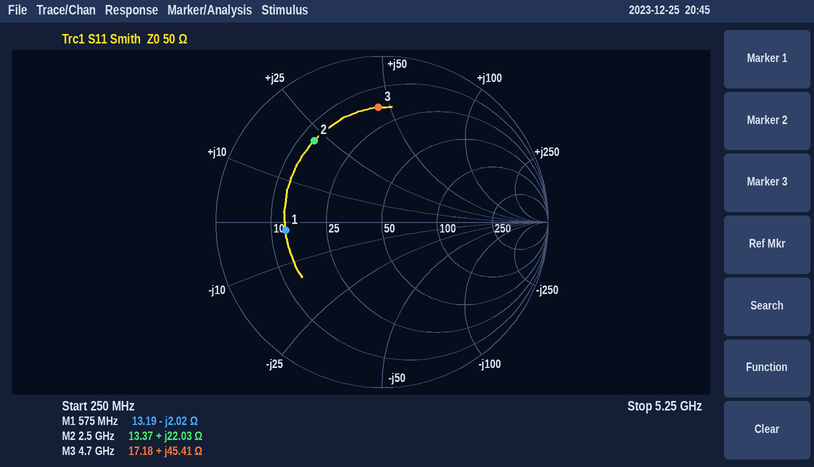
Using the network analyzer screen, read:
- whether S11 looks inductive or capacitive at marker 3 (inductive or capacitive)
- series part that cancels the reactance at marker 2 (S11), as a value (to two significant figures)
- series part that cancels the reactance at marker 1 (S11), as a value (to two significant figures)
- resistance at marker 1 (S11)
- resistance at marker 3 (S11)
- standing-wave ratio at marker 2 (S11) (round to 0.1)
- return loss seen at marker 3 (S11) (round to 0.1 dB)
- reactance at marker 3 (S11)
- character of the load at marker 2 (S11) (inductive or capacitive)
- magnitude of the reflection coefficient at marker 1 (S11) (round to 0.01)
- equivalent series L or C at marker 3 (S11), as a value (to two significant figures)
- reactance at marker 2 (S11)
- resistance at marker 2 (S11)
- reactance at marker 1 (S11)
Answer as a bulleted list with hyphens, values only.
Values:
- inductive
- 2.9 pF
- 560 pH
- 13.19 Ω
- 17.18 Ω
- 4.5
- 3.2 dB
- +45.41 Ω
- inductive
- 0.58
- 1.5 nH
- +22.03 Ω
- 13.37 Ω
- -2.02 Ω
